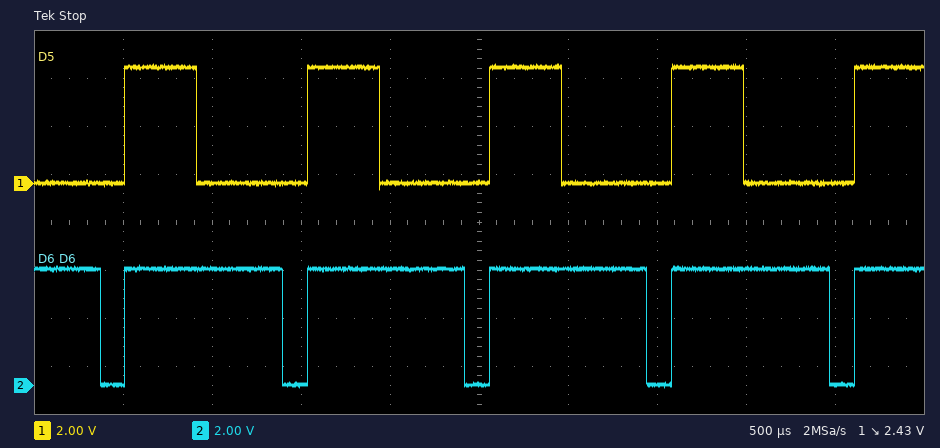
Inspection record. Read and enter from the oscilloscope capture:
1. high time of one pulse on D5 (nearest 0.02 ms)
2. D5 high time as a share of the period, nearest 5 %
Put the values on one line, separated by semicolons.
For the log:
0.40 ms; 40 %
